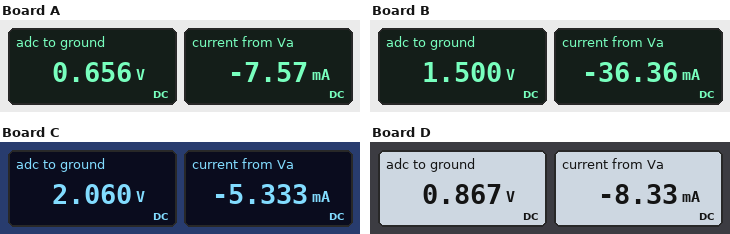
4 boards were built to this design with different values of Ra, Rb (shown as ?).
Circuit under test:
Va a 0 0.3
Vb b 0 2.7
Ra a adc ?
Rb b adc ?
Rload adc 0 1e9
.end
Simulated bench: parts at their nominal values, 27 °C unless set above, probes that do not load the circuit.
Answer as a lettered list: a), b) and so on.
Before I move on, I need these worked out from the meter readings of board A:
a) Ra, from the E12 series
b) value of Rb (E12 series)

a) 47 Ω
b) 270 Ω
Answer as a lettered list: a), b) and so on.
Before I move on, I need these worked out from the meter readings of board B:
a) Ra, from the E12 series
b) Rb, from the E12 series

a) 33 Ω
b) 33 Ω
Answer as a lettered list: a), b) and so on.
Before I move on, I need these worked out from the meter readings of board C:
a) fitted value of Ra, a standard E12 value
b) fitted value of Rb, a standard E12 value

a) 330 Ω
b) 120 Ω
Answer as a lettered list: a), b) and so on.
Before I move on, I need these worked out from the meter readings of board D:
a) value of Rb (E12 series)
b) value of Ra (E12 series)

a) 220 Ω
b) 68 Ω
